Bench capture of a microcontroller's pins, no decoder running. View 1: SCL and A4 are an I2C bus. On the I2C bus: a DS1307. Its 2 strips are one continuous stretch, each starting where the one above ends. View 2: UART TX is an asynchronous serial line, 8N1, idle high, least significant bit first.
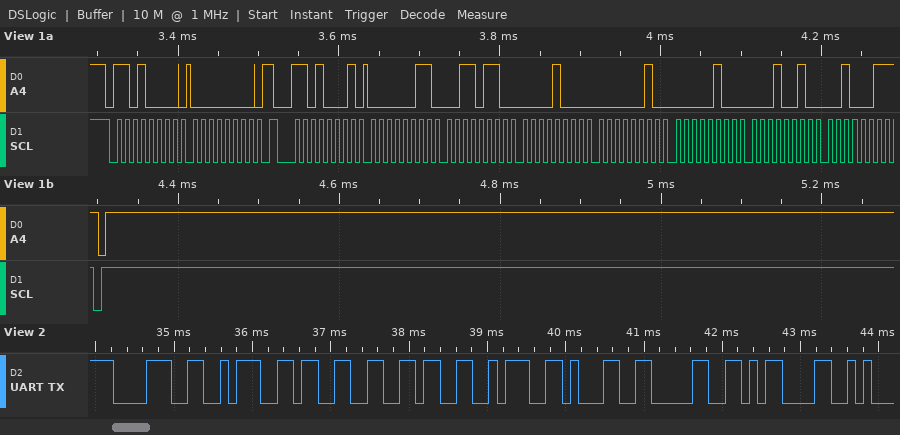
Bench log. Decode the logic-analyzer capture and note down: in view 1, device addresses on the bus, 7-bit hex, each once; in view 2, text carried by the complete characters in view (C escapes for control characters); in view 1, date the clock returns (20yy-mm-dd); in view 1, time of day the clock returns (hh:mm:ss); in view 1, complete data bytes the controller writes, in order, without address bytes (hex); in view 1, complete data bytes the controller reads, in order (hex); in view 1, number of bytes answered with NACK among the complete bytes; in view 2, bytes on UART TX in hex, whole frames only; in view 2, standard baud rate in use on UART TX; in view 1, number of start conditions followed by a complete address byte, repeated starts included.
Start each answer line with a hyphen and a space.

- 0x68
- "8:36:10\r"
- 2023-12-04
- 08:36:03
- 00
- 03 36 08 02 04 12 23
- 1
- 0x38 0x3A 0x33 0x36 0x3A 0x31 0x30 0x0D
- 9600 baud
- 2
